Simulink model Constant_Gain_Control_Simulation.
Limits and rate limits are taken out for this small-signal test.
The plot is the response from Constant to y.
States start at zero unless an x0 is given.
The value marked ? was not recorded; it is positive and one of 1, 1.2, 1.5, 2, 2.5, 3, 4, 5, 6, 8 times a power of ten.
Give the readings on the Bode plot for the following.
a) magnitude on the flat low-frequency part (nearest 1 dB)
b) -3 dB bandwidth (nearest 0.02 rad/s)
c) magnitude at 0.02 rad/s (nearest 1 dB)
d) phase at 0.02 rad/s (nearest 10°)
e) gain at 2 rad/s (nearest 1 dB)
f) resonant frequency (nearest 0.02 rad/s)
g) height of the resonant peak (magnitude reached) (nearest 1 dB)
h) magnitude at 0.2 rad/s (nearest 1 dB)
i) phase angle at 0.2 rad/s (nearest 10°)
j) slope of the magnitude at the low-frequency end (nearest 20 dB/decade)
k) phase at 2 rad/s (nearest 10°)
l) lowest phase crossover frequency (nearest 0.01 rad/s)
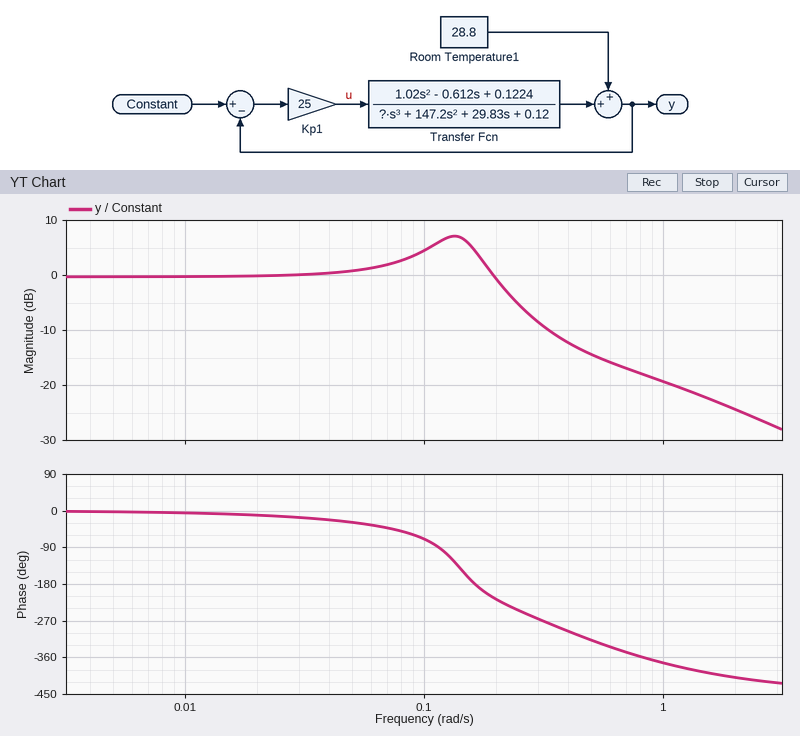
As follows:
0 dB
0.22 rad/s
0 dB
-10°
-24 dB
0.14 rad/s
7 dB
-1 dB
-220°
0 dB/decade
-410°
0.16 rad/s
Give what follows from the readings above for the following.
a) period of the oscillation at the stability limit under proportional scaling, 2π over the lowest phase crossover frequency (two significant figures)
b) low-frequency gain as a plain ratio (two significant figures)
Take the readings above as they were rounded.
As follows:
39 s
1.0
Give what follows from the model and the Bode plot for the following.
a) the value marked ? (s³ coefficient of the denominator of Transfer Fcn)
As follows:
200
